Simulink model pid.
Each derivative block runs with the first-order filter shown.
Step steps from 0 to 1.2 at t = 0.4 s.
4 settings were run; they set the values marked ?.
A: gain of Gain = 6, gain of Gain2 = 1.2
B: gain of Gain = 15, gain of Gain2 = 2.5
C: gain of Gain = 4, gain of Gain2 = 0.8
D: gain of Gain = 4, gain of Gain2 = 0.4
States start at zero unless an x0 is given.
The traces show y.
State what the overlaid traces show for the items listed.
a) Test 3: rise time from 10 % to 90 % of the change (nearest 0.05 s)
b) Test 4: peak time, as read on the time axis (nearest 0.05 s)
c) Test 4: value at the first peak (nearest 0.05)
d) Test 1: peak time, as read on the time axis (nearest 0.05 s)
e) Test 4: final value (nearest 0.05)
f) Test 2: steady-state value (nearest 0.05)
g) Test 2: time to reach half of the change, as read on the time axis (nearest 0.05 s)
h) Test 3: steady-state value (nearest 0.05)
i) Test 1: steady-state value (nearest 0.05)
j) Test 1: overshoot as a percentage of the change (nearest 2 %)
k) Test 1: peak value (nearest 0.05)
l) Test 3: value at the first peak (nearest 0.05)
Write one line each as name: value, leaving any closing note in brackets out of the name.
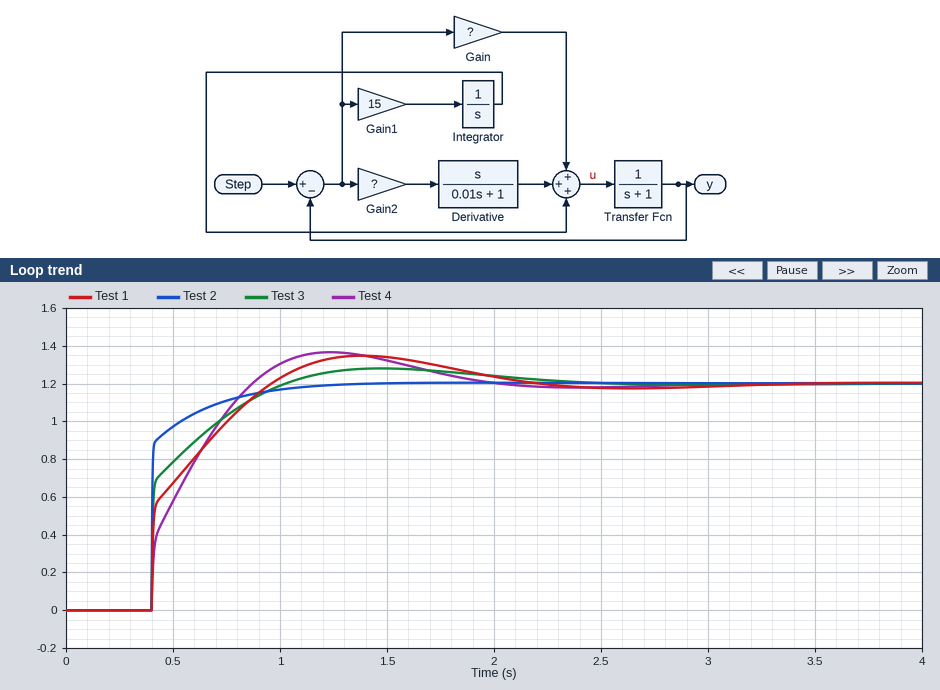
Test 3: rise time from 10 % to 90 % of the change: 0.40 s
Test 4: peak time, as read on the time axis: 1.25 s
Test 4: value at the first peak: 1.35
Test 1: peak time, as read on the time axis: 1.40 s
Test 4: final value: 1.20
Test 2: steady-state value: 1.20
Test 2: time to reach half of the change, as read on the time axis: 0.40 s
Test 3: steady-state value: 1.20
Test 1: steady-state value: 1.20
Test 1: overshoot as a percentage of the change: 12 %
Test 1: peak value: 1.35
Test 3: value at the first peak: 1.30
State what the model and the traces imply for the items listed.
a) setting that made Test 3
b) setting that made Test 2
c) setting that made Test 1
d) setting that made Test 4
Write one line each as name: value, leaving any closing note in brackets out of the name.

setting that made Test 3: A
setting that made Test 2: B
setting that made Test 1: C
setting that made Test 4: D
